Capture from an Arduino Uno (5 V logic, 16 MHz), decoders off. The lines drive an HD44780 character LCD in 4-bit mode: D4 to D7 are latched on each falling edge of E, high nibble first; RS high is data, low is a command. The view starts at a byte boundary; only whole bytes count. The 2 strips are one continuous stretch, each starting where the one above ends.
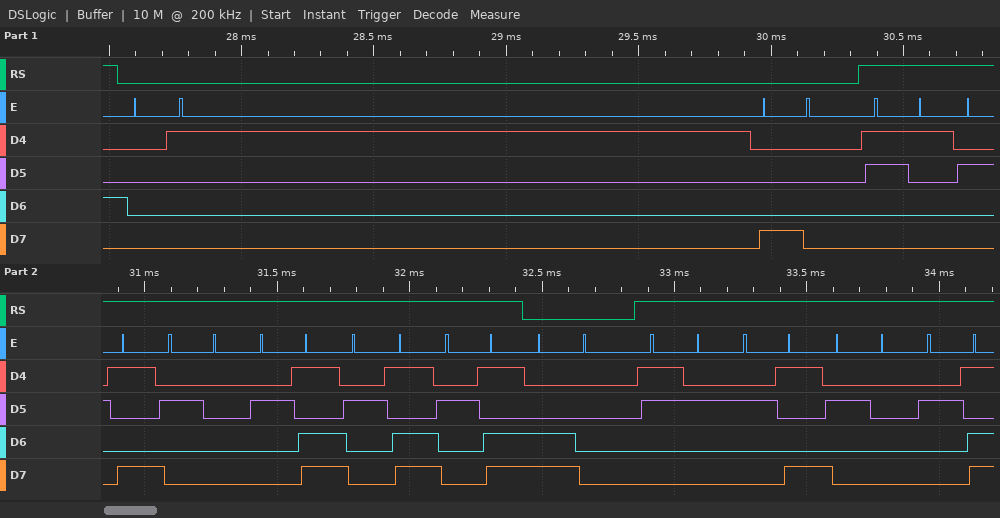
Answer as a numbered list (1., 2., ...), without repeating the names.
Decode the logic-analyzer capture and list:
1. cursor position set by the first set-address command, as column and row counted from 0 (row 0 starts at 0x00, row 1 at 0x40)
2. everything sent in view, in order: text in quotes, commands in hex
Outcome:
1. column 0, row 0
2. 0x01 0x80 "1) ---" 0xC0 "2) -"
